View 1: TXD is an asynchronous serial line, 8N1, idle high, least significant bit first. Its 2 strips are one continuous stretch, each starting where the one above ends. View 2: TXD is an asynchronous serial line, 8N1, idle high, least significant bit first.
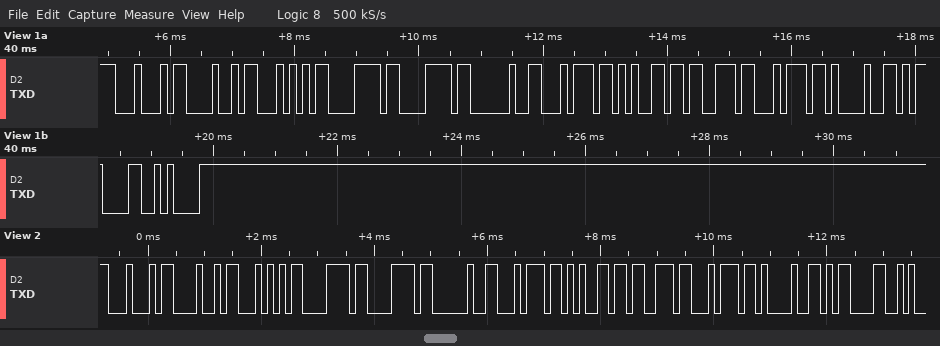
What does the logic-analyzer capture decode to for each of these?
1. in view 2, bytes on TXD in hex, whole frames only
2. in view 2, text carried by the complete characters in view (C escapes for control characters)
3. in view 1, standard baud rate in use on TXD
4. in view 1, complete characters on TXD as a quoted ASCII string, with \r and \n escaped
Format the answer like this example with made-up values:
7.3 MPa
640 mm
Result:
44 48 54 78 78 20 74 65 73 74 21 0D
"DHTxx test!\r"
9600 baud
"DHTxx test!\r\n"
